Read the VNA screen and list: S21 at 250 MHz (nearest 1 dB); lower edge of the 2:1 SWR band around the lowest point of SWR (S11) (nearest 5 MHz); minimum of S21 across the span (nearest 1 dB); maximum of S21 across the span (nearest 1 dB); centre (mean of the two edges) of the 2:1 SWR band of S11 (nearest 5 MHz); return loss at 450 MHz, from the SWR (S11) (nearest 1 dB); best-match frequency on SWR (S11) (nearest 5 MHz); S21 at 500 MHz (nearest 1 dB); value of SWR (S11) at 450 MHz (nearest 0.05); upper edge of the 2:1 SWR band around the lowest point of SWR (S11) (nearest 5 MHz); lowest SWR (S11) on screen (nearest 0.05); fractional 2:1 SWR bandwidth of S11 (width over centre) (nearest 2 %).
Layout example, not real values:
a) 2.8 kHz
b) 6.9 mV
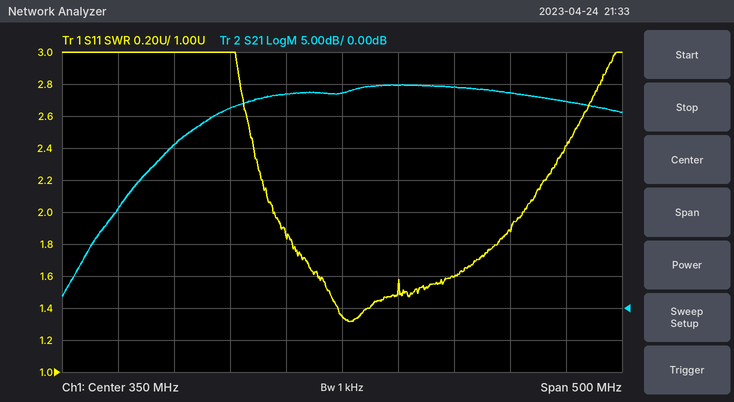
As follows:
a) 31 dB
b) 290 MHz
c) 2 dB
d) 35 dB
e) 400 MHz
f) 13 dB
g) 355 MHz
h) 34 dB
i) 1.60
j) 510 MHz
k) 1.30
l) 56 %
